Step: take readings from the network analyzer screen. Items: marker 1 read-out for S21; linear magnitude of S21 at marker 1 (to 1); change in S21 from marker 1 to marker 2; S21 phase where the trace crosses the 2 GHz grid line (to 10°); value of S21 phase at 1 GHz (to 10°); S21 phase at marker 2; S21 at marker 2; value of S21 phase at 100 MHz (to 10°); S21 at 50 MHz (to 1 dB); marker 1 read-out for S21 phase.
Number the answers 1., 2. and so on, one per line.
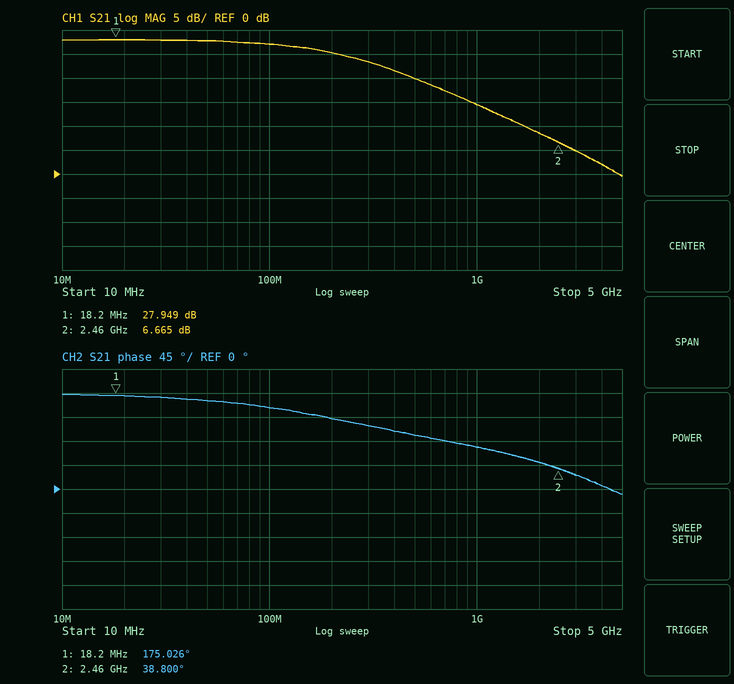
1. 27.949 dB
2. 25
3. -21.284 dB
4. 50°
5. 80°
6. 38.800°
7. 6.665 dB
8. 150°
9. 28 dB
10. 175.026°
